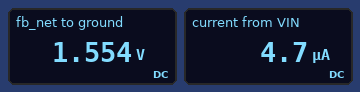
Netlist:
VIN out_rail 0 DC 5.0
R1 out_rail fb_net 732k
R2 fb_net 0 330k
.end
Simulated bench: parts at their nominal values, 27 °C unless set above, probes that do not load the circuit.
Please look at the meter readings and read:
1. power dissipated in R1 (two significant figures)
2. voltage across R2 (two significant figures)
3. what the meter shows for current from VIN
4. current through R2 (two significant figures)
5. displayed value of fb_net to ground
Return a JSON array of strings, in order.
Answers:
["16 µW", "1.6 V", "4.7 µA", "4.7 µA", "1.554 V"]
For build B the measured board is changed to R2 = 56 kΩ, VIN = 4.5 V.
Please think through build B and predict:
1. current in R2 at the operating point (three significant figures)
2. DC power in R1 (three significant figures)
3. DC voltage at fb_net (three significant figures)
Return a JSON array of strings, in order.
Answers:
["5.71 µA", "23.9 µW", "320 mV"]
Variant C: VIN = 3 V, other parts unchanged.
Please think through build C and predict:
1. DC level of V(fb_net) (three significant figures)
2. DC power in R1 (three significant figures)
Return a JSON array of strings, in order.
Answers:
["932 mV", "5.84 µW"]
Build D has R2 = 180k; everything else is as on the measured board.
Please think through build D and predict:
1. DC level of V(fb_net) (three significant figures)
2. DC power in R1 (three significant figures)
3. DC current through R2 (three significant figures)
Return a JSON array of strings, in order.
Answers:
["987 mV", "22.0 µW", "5.48 µA"]
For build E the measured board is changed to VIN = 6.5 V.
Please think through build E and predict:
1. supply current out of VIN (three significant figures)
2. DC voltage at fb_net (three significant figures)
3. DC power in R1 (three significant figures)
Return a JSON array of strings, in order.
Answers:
["6.12 µA", "2.02 V", "27.4 µW"]
